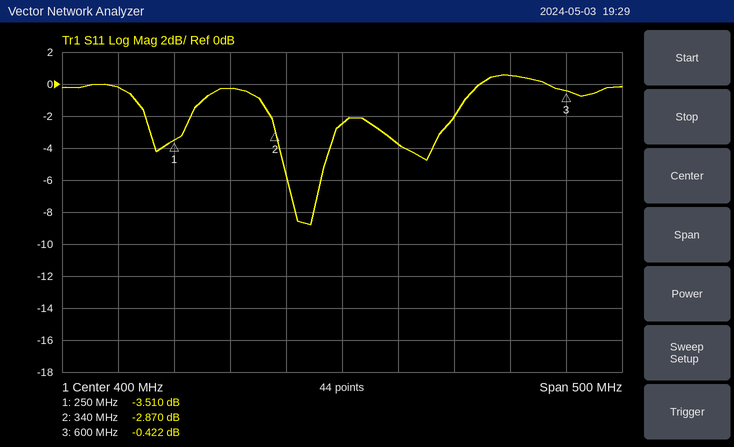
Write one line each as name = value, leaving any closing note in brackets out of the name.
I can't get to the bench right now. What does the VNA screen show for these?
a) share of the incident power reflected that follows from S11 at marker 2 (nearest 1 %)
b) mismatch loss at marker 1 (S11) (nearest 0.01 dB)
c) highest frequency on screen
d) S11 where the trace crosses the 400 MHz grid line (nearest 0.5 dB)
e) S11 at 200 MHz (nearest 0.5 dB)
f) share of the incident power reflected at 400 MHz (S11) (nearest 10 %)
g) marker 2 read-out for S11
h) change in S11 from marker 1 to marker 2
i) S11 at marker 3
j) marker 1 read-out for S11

share of the incident power reflected that follows from S11 at marker 2 = 52 %
mismatch loss at marker 1 (S11) = 2.56 dB
highest frequency on screen = 650 MHz
S11 where the trace crosses the 400 MHz grid line = -2.5 dB
S11 at 200 MHz = 0.0 dB
share of the incident power reflected at 400 MHz (S11) = 60 %
marker 2 read-out for S11 = -2.870 dB
change in S11 from marker 1 to marker 2 = 0.640 dB
S11 at marker 3 = -0.422 dB
marker 1 read-out for S11 = -3.510 dB
